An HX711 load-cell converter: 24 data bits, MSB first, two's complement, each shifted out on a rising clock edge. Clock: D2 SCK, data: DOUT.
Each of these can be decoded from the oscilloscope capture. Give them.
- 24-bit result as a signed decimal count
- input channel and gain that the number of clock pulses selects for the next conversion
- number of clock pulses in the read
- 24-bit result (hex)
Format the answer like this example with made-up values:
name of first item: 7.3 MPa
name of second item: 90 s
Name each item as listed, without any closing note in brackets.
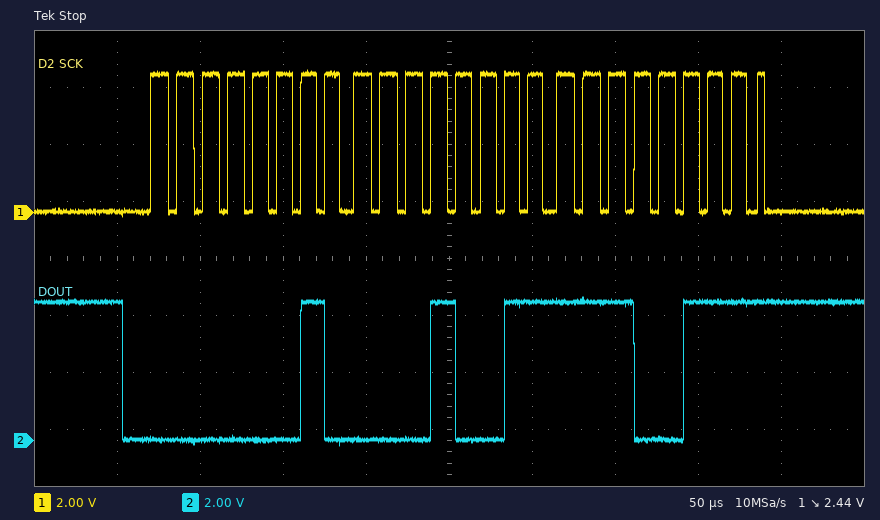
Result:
24-bit result as a signed decimal count: 136167
input channel and gain that the number of clock pulses selects for the next conversion: channel A, gain 128
number of clock pulses in the read: 25
24-bit result: 0x0213E7
